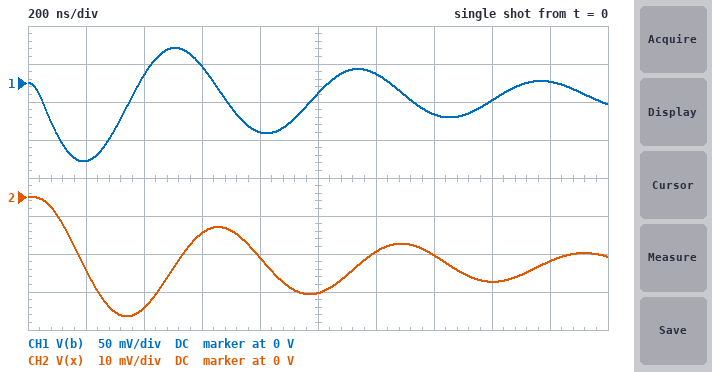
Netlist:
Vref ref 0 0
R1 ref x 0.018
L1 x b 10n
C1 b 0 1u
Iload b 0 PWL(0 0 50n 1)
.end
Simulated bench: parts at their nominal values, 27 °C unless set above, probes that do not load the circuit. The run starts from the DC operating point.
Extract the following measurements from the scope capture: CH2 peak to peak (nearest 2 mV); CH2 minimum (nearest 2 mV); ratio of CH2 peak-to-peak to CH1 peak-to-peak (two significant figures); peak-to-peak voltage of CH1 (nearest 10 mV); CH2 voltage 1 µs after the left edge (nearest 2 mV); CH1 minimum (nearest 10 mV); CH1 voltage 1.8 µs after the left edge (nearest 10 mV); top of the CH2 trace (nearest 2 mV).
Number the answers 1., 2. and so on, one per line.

1. 32 mV
2. -32 mV
3. 0.21
4. 150 mV
5. -26 mV
6. -100 mV
7. 0 V
8. 0 V
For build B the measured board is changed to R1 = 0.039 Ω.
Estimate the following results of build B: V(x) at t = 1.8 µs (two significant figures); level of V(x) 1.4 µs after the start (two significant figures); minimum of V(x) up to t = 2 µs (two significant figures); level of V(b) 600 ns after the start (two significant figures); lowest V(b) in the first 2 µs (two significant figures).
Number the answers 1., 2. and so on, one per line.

1. -39 mV
2. -37 mV
3. -60 mV
4. -11 mV
5. -110 mV
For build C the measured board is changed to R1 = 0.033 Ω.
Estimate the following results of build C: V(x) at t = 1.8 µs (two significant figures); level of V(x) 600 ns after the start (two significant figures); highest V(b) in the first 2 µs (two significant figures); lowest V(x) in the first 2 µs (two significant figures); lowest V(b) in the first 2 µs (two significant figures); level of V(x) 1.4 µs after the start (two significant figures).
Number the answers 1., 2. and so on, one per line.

1. -33 mV
2. -24 mV
3. 11 mV
4. -52 mV
5. -110 mV
6. -31 mV
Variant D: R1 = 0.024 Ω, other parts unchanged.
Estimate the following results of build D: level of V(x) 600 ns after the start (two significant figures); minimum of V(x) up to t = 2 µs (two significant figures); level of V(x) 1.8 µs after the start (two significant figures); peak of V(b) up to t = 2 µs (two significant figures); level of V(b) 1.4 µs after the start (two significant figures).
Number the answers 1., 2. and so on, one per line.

1. -15 mV
2. -40 mV
3. -23 mV
4. 31 mV
5. -38 mV
